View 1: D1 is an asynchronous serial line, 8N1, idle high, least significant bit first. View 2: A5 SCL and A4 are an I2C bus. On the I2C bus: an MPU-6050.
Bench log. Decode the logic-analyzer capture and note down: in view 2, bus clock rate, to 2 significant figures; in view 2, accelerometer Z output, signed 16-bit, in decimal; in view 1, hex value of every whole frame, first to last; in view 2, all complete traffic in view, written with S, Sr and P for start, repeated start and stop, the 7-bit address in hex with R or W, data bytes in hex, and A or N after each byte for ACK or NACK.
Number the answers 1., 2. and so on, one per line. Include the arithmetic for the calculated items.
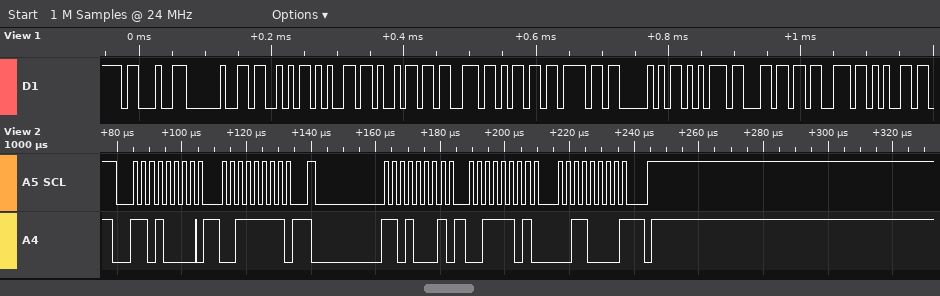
1. 400 kHz
2. 0x3D30 = 15664
3. 23 20 53 65 69 73 6D 6F 50 75 6C 73 65
4. S 68W A 3F A Sr 68R A 3D A 30 N P
